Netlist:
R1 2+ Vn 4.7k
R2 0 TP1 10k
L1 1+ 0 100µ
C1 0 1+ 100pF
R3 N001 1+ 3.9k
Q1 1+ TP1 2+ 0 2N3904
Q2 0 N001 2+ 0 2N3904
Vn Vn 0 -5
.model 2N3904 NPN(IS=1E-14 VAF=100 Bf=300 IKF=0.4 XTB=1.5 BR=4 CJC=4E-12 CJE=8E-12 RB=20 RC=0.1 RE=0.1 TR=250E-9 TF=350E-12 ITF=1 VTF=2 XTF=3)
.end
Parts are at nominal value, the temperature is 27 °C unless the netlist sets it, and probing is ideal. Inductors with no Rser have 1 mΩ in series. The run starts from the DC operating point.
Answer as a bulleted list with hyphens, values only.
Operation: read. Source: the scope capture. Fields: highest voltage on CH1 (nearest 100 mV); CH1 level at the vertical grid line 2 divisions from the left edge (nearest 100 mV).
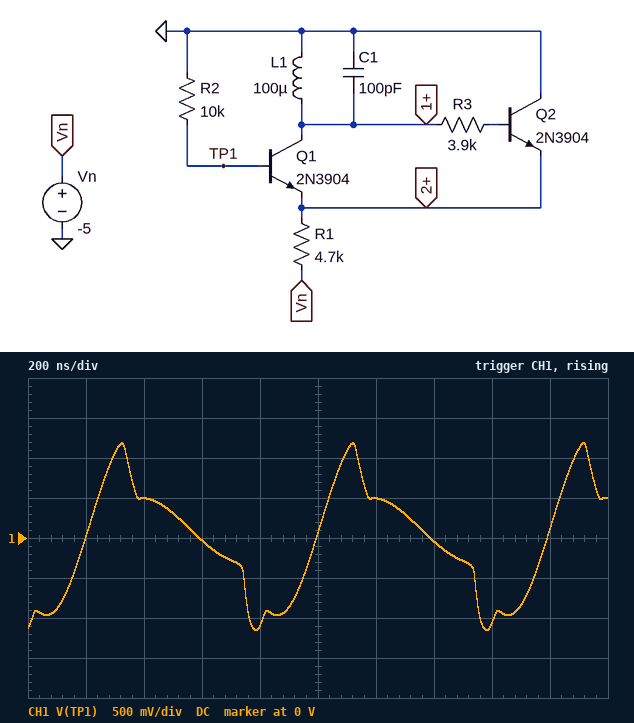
- 1.2 V
- 500 mV
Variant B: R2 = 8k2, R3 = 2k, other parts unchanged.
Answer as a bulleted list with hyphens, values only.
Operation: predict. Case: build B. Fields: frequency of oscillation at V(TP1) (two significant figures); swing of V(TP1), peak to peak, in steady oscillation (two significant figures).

- 1.2 MHz
- 2.1 V
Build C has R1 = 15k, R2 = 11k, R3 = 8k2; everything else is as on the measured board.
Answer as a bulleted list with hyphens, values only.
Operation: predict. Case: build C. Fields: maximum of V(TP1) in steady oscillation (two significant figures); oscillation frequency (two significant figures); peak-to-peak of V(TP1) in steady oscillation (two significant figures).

- 620 mV
- 1.4 MHz
- 1.4 V
